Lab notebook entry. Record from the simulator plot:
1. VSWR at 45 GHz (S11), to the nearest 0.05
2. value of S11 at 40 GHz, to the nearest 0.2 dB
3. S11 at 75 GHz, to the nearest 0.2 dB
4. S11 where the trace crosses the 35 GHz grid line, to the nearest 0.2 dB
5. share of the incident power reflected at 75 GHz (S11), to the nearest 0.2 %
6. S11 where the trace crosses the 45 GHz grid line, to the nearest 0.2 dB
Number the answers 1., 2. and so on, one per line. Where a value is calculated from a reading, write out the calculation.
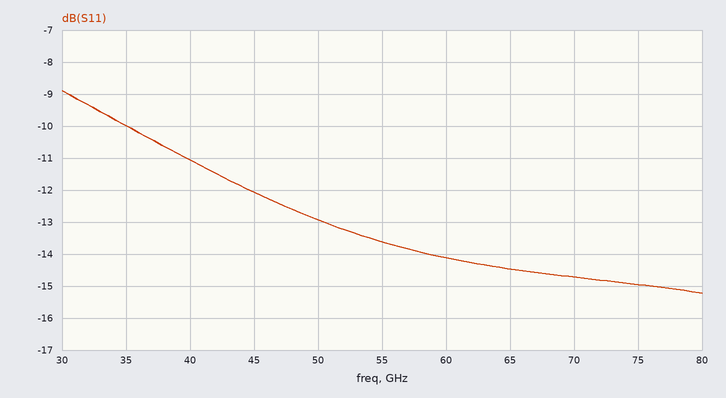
1. |Γ| = 10^(-12/20) = 0.2512; VSWR = (1 + 0.2512)/(1 − 0.2512) ≈ 1.67, so 1.65 to the nearest 0.05
2. -11.0 dB
3. -15.0 dB
4. -10.0 dB
5. 10^(-15/10) ≈ 3.2 %
6. -12.0 dB
